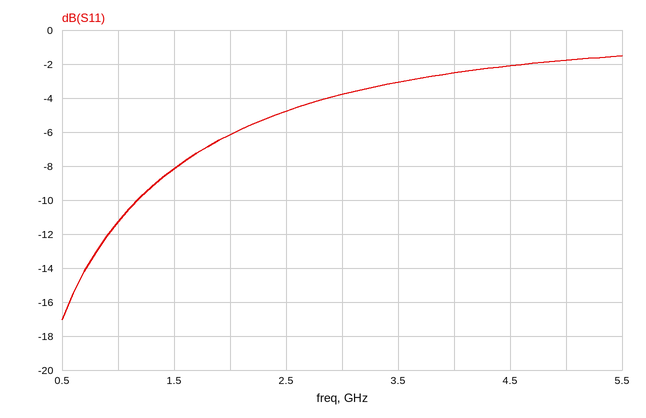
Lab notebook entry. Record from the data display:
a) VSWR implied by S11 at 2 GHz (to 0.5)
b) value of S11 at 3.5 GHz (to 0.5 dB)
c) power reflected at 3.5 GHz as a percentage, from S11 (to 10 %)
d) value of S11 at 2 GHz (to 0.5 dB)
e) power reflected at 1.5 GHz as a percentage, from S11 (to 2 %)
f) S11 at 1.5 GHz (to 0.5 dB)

3.0
-3.0 dB
50 %
-6.0 dB
16 %
-8.0 dB
